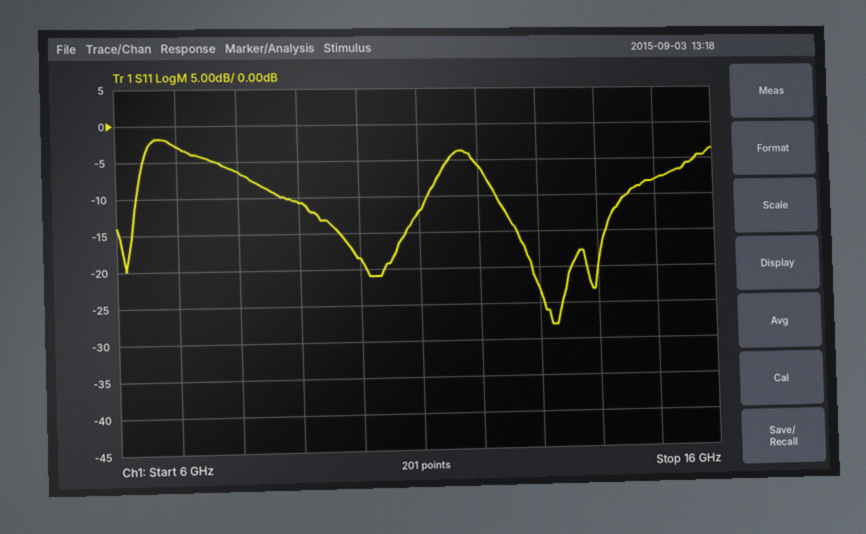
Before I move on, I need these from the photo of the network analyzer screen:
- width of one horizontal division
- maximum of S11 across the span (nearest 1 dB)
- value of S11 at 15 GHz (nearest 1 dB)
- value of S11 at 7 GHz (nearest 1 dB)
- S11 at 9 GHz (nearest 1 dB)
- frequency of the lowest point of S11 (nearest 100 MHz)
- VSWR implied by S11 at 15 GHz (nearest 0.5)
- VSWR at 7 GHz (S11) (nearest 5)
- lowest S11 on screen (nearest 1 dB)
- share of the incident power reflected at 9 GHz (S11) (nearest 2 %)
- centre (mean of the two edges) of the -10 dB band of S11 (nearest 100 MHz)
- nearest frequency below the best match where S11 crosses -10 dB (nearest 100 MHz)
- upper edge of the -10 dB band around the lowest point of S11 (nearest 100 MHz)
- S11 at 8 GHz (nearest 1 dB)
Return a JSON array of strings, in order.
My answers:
["1 GHz", "-2 dB", "-8 dB", "-3 dB", "-11 dB", "13.2 GHz", "2.5", "5", "-28 dB", "8 %", "13.4 GHz", "12.3 GHz", "14.5 GHz", "-6 dB"]
